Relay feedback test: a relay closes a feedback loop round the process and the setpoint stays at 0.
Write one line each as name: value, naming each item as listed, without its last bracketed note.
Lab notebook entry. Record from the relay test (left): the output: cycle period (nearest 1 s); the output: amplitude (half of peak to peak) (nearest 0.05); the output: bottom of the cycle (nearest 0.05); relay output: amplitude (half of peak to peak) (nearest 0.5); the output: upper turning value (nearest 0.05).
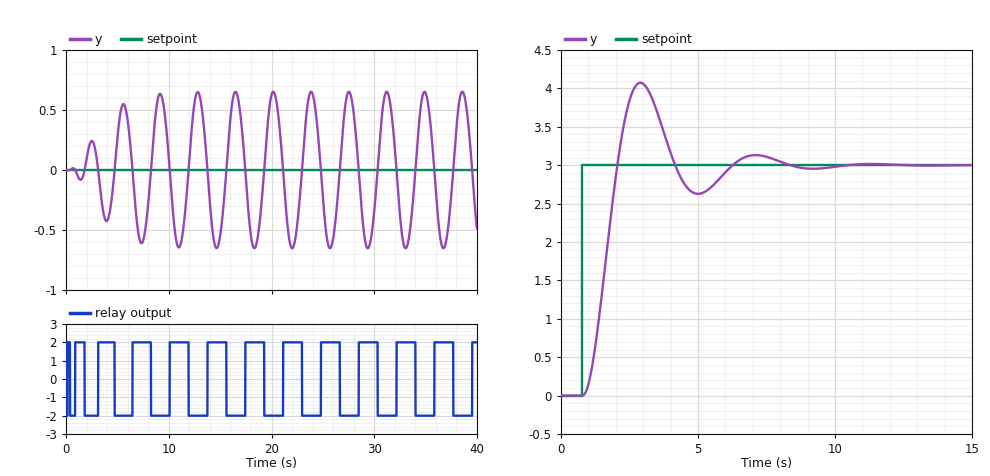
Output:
the output: cycle period: 4 s
the output: amplitude (half of peak to peak): 0.65
the output: bottom of the cycle: -0.65
relay output: amplitude (half of peak to peak): 2.0
the output: upper turning value: 0.65
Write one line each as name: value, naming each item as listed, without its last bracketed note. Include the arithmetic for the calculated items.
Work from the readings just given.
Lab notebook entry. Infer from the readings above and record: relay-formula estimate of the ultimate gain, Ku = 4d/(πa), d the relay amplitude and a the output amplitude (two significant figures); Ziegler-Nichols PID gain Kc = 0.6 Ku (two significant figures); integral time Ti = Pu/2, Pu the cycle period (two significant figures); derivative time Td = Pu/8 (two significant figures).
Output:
relay-formula estimate of the ultimate gain, Ku = 4d/(πa), d the relay amplitude and a the output amplitude: 4 × 2 / (π × 0.65) = 3.9
Ziegler-Nichols PID gain Kc = 0.6 Ku: 0.6 × 3.9 = 2.3
integral time Ti = Pu/2, Pu the cycle period: 4 / 2 = 2.0 s
derivative time Td = Pu/8: 4 / 8 = 0.50 s
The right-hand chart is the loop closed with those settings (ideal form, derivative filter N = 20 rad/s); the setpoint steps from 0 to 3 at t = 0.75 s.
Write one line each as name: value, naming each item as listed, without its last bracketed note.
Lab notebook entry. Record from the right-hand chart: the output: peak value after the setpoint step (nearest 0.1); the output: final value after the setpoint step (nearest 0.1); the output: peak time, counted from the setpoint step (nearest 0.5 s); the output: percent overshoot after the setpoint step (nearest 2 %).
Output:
the output: peak value after the setpoint step: 4.1
the output: final value after the setpoint step: 3.0
the output: peak time, counted from the setpoint step: 2.0 s
the output: percent overshoot after the setpoint step: 36 %
